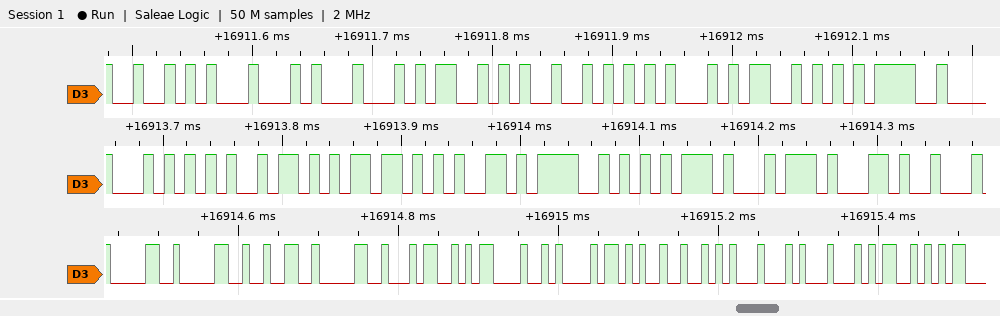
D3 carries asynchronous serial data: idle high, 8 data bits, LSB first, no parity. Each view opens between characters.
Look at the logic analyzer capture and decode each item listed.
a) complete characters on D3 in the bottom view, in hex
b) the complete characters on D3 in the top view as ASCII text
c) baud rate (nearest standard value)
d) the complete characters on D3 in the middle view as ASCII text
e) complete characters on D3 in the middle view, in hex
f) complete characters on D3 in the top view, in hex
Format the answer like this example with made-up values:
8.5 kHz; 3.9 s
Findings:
30, 30, 32, 30, 34, 0D, 0A, 2B, 52, 44, 44, 53; "RDDSRES="; 115200 baud; "TimeOut,"; 54, 69, 6D, 65, 4F, 75, 74, 2C; 52, 44, 44, 53, 52, 45, 53, 3D
